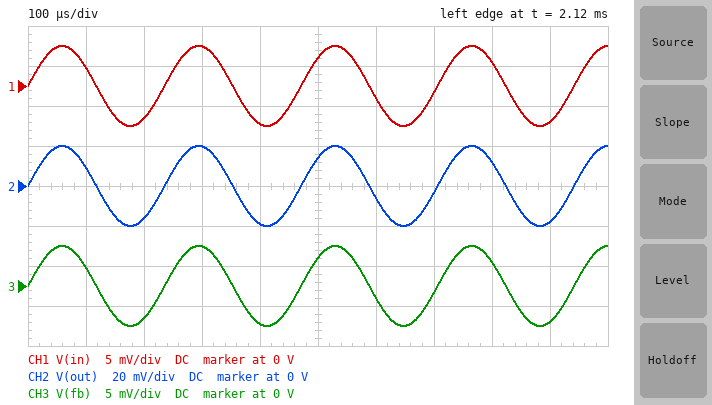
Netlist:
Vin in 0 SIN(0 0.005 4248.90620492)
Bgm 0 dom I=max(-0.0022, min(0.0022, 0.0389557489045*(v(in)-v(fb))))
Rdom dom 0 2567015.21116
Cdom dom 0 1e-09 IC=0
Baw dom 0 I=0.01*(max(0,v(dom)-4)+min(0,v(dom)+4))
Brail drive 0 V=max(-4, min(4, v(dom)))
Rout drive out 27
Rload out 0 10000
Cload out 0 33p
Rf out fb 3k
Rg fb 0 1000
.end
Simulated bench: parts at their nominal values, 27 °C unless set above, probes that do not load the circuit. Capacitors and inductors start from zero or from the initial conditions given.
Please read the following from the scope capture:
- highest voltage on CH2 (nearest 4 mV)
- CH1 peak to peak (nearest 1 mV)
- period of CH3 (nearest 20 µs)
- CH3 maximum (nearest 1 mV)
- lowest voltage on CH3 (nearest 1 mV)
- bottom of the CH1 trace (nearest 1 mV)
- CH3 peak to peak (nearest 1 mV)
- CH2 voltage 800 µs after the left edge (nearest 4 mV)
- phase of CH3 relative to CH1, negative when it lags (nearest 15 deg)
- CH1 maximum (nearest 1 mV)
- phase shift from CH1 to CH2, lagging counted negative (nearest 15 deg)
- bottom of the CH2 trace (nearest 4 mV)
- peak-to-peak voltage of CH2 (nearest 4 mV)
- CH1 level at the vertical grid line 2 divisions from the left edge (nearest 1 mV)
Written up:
20 mV
10 mV
240 µs
5 mV
-5 mV
-5 mV
10 mV
12 mV
0 deg
5 mV
0 deg
-20 mV
40 mV
-4 mV
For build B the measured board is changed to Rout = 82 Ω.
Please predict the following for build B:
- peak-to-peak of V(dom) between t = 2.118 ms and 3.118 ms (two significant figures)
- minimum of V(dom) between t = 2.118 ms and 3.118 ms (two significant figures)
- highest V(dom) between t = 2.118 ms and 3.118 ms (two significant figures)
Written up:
41 mV
-21 mV
21 mV
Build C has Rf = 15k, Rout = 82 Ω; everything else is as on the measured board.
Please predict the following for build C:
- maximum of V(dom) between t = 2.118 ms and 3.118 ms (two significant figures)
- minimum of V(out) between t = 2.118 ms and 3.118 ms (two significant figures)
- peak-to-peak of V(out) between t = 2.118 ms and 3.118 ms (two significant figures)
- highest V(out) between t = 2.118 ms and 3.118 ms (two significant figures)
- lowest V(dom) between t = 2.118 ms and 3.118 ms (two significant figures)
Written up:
81 mV
-80 mV
160 mV
80 mV
-81 mV
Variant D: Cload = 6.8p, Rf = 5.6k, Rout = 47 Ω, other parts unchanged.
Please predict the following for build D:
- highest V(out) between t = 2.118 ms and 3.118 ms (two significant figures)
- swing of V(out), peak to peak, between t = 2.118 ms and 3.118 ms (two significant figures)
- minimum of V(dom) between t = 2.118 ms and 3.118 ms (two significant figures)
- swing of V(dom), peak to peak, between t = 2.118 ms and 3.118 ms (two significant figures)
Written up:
33 mV
66 mV
-33 mV
67 mV
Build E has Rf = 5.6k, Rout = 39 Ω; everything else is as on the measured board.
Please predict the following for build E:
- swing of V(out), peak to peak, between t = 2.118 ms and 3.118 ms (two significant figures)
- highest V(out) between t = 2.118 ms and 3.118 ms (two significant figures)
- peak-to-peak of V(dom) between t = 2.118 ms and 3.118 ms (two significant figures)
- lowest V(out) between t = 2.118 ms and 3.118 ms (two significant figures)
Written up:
66 mV
33 mV
67 mV
-33 mV
